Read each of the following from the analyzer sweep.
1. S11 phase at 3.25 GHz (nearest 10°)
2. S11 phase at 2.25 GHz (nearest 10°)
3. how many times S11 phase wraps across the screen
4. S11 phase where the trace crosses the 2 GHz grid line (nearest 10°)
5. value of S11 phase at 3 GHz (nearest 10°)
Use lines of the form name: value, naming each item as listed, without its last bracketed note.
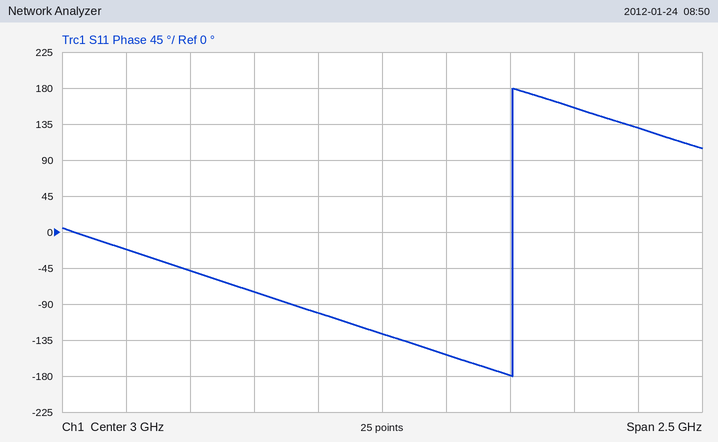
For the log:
S11 phase at 3.25 GHz: -150°
S11 phase at 2.25 GHz: -50°
how many times S11 phase wraps across the screen: 1
S11 phase where the trace crosses the 2 GHz grid line: -20°
value of S11 phase at 3 GHz: -130°
